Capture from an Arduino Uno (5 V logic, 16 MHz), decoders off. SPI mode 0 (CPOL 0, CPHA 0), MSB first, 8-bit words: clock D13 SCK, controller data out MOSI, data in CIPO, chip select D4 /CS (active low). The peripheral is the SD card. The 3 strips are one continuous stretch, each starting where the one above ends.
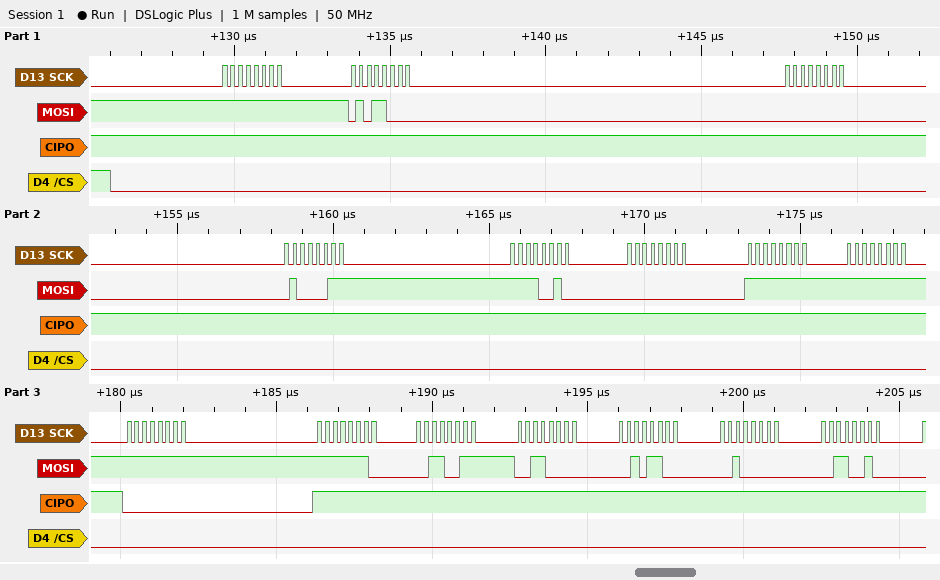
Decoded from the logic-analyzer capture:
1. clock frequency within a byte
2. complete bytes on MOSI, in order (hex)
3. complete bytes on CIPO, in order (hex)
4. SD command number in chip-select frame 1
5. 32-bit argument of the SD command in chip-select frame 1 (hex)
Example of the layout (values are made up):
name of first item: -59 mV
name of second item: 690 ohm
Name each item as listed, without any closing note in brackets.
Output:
clock frequency within a byte: 4 MHz
complete bytes on MOSI, in order: FF 58 00 43 F2 00 FF FF FF FE 33 30 2C 20 32
complete bytes on CIPO, in order: FF FF FF FF FF FF FF FF 00 FF FF FF FF FF FF
SD command number in chip-select frame 1: CMD24
32-bit argument of the SD command in chip-select frame 1: 0x0043F200
